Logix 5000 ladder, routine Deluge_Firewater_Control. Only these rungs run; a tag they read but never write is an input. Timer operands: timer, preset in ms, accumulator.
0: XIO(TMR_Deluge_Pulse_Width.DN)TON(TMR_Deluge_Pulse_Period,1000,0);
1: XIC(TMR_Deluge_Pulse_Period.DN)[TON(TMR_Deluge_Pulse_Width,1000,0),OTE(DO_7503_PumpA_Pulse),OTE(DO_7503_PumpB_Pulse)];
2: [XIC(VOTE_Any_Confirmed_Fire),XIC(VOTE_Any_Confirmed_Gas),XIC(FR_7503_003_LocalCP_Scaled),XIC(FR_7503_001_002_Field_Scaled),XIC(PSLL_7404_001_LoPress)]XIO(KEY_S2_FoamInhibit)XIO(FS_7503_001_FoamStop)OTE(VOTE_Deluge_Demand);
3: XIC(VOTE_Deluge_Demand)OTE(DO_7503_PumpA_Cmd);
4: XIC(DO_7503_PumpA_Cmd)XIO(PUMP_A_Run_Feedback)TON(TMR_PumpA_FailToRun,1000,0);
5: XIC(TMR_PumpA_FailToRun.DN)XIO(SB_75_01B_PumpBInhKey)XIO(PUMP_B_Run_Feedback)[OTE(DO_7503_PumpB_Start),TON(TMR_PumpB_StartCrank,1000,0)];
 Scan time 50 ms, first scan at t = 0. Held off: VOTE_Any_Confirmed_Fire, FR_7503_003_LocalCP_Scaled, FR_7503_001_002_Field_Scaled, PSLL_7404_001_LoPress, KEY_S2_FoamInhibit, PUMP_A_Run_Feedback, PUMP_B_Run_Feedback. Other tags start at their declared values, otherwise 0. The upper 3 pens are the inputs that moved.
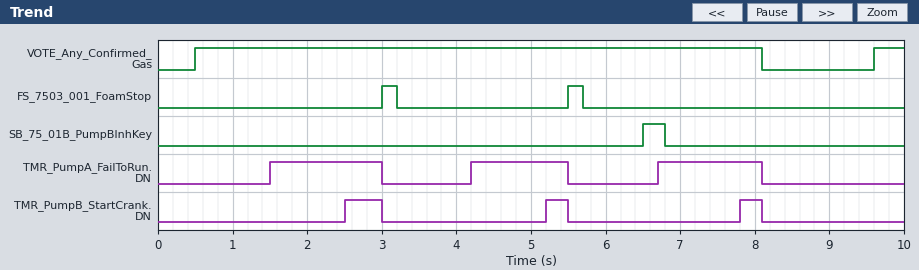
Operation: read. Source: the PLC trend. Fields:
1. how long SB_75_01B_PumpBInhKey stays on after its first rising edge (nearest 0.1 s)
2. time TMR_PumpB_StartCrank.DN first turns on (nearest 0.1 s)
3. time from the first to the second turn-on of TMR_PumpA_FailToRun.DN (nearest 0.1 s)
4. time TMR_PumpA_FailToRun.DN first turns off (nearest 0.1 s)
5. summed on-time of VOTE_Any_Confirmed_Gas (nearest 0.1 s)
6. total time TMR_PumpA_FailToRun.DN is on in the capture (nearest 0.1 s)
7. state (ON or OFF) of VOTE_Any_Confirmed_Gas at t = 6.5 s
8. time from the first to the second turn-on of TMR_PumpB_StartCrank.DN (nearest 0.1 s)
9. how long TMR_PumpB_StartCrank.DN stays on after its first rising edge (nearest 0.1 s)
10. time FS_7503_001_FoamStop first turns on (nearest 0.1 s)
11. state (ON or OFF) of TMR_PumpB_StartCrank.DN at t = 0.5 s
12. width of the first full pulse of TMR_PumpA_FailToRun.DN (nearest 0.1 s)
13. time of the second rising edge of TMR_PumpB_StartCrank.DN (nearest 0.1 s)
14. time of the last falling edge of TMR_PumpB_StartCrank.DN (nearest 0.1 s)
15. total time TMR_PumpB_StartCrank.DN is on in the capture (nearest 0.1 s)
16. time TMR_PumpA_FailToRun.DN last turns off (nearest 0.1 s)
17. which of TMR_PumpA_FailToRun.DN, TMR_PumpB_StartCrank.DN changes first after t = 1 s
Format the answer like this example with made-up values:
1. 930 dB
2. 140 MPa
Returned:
1. 0.3 s
2. 2.5 s
3. 2.7 s
4. 3.0 s
5. 8.0 s
6. 4.2 s
7. ON
8. 2.7 s
9. 0.5 s
10. 3.0 s
11. OFF
12. 1.5 s
13. 5.2 s
14. 8.1 s
15. 1.1 s
16. 8.1 s
17. TMR_PumpA_FailToRun.DN
